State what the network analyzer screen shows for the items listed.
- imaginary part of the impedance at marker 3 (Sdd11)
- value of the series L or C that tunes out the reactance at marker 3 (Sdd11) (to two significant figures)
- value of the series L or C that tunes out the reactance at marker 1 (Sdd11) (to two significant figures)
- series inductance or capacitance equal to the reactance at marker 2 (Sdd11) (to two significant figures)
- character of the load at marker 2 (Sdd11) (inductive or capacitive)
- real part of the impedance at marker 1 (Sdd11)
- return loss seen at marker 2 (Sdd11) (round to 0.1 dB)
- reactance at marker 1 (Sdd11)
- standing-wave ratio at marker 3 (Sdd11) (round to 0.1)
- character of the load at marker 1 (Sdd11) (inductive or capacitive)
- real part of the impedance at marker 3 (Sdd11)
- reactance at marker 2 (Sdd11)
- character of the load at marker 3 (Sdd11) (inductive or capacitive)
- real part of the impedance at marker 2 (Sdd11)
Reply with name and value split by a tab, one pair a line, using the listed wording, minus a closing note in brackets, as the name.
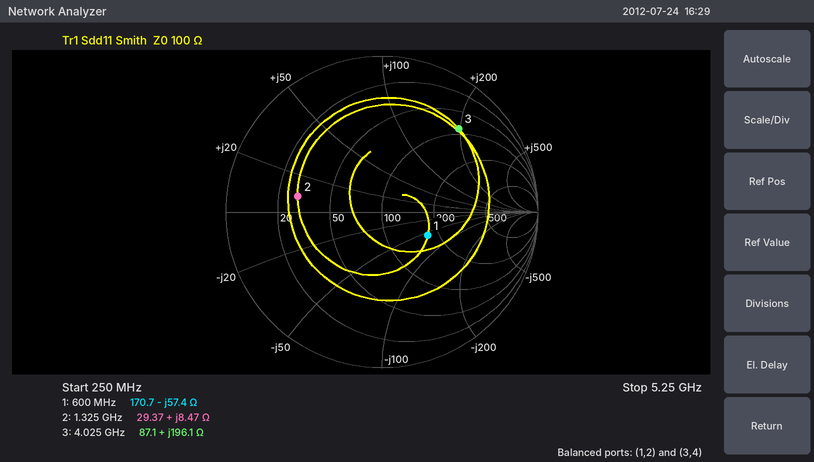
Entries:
imaginary part of the impedance at marker 3	+196.1 Ω
value of the series L or C that tunes out the reactance at marker 3 (Sdd11)	200 fF
value of the series L or C that tunes out the reactance at marker 1 (Sdd11)	15 nH
series inductance or capacitance equal to the reactance at marker 2 (Sdd11)	1.0 nH
character of the load at marker 2 (Sdd11)	inductive
real part of the impedance at marker 1	170.7 Ω
return loss seen at marker 2 (Sdd11)	5.2 dB
reactance at marker 1	-57.4 Ω
standing-wave ratio at marker 3 (Sdd11)	6.3
character of the load at marker 1 (Sdd11)	capacitive
real part of the impedance at marker 3	87.1 Ω
reactance at marker 2	+8.47 Ω
character of the load at marker 3 (Sdd11)	inductive
real part of the impedance at marker 2	29.37 Ω
